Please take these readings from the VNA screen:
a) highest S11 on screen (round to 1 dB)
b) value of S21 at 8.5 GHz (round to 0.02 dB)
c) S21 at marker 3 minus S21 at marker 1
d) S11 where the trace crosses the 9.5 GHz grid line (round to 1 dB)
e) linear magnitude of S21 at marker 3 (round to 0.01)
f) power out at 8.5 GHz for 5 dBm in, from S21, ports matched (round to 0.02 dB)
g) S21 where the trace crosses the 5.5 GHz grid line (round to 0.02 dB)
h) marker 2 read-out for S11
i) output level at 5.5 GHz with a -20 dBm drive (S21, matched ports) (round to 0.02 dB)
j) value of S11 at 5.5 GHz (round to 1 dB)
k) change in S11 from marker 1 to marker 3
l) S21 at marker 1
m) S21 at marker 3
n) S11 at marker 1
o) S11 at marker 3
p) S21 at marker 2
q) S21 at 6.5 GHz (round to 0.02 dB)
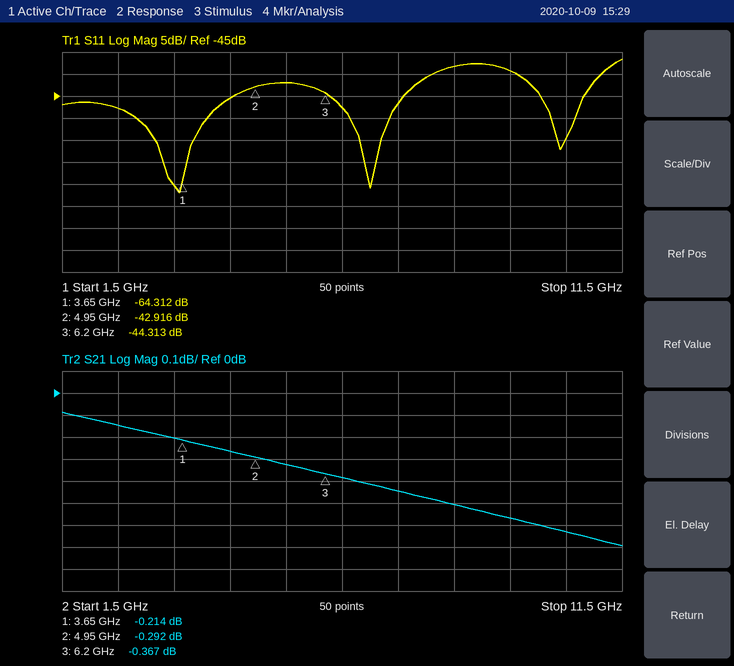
-37 dB
-0.50 dB
-0.153 dB
-39 dB
0.96
4.50 dBm
-0.32 dB
-42.916 dB
-20.32 dBm
-42 dB
19.999 dB
-0.214 dB
-0.367 dB
-64.312 dB
-44.313 dB
-0.292 dB
-0.38 dB
